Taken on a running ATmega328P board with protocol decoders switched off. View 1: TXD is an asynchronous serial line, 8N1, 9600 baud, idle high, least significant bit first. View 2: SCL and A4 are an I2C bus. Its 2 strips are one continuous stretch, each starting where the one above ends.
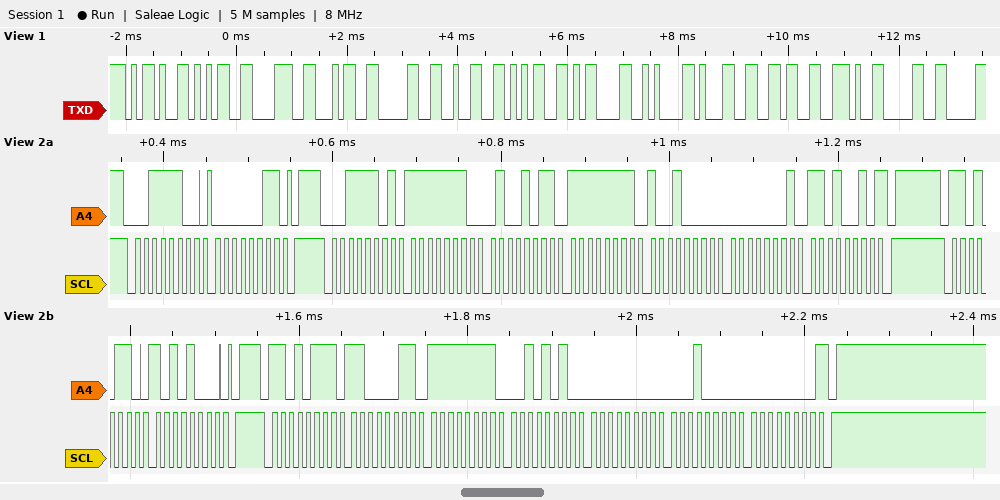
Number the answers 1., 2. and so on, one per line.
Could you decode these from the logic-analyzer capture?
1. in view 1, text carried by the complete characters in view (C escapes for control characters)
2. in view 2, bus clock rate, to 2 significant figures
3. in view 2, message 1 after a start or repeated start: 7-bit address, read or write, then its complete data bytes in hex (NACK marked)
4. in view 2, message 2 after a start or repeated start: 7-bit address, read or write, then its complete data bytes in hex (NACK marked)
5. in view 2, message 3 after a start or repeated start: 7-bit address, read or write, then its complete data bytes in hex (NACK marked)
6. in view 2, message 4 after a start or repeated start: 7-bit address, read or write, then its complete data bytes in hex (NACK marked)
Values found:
1. "-584025\r\n16.0"
2. 100 kHz
3. 0x1E write: 03
4. 0x1E read: FE 4B FF 90 01 D2 NACK
5. 0x6B write: A8
6. 0x6B read: C3 FF 2A 00 10 00 NACK
